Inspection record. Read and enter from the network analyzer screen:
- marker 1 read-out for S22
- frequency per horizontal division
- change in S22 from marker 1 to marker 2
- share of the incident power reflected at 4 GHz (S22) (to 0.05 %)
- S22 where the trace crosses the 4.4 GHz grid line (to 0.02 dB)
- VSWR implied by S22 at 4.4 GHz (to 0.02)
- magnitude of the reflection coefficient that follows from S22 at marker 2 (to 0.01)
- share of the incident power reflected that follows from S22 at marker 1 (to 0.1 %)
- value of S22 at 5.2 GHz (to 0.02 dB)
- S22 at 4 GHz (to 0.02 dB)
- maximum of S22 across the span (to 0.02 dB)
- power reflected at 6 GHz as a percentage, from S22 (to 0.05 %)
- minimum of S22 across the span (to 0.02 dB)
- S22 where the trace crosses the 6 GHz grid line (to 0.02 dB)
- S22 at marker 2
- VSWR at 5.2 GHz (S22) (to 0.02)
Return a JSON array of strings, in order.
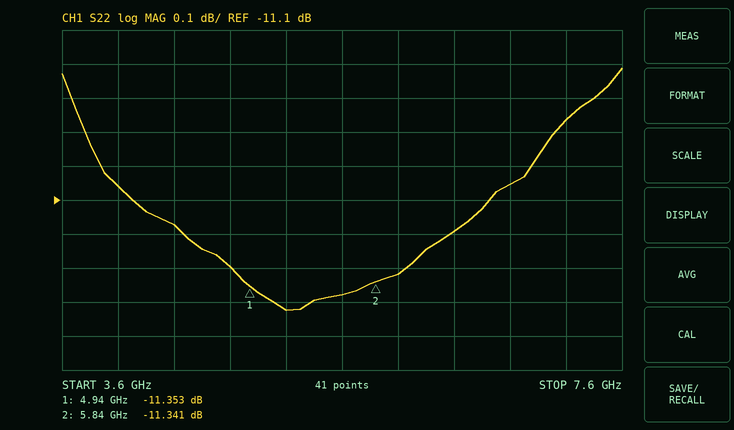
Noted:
["-11.353 dB", "400 MHz", "0.012 dB", "7.85 %", "-11.18 dB", "1.76", "0.27", "7.3 %", "-11.42 dB", "-11.06 dB", "-10.72 dB", "7.40 %", "-11.42 dB", "-11.32 dB", "-11.341 dB", "1.74"]
